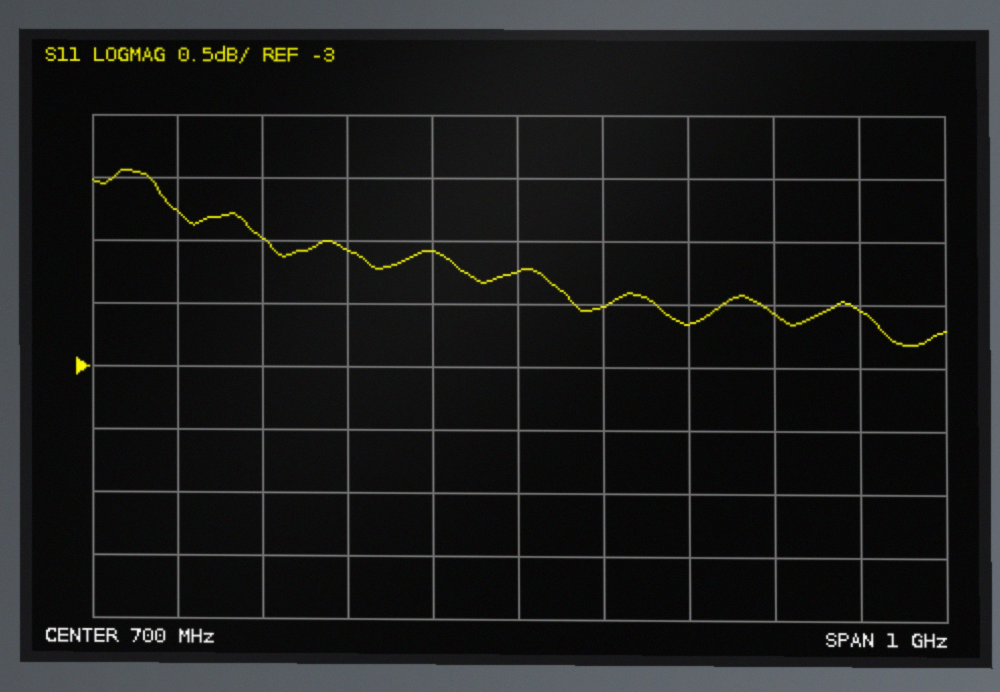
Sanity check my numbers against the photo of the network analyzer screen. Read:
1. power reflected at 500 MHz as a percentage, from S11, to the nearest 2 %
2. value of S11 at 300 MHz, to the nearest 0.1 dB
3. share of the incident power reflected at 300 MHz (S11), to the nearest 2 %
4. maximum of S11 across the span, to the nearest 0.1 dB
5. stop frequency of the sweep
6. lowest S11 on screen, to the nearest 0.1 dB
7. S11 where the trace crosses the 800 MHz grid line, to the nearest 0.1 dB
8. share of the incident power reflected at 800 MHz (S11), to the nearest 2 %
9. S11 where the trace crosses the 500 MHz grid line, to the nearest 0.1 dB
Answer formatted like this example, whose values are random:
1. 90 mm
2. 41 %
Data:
1. 62 %
2. -1.8 dB
3. 66 %
4. -1.4 dB
5. 1.2 GHz
6. -2.8 dB
7. -2.5 dB
8. 56 %
9. -2.1 dB
